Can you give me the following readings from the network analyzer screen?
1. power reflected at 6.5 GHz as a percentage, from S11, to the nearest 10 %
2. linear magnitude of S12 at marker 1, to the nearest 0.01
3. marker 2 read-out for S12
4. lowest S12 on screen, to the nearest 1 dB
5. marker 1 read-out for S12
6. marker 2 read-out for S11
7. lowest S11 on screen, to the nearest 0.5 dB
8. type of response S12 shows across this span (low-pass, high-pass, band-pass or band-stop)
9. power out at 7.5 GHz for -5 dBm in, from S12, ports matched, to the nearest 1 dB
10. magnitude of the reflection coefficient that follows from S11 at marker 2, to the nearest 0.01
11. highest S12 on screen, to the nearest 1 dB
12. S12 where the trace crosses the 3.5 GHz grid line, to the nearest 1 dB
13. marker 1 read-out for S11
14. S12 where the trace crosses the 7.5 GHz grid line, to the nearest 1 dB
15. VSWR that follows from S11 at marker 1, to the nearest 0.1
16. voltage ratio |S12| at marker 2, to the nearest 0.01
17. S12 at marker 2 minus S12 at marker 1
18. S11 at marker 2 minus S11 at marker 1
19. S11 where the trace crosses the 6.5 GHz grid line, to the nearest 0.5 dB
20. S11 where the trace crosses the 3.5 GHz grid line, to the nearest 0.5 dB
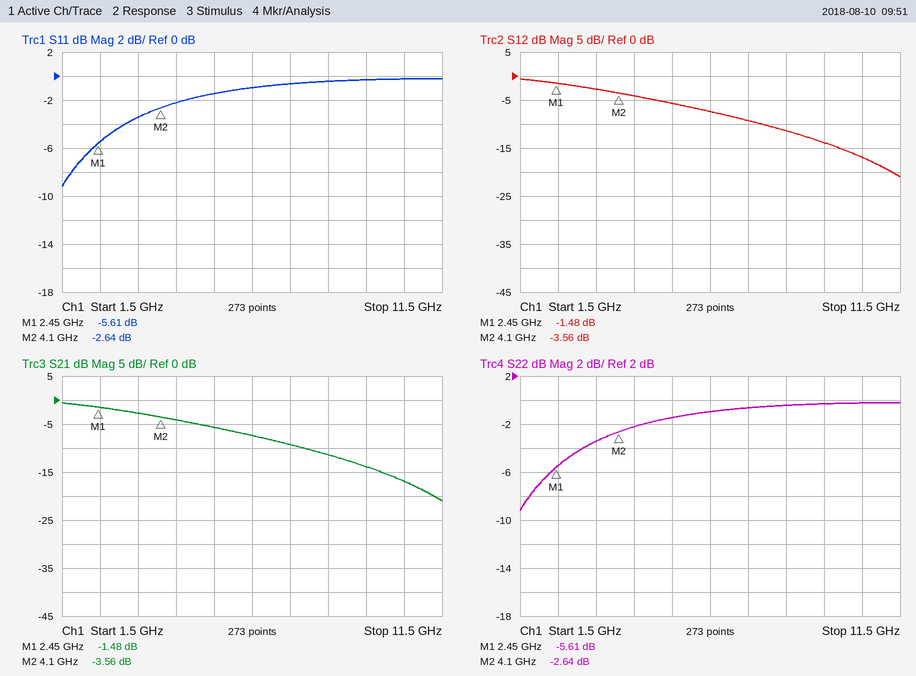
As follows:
80 %
0.84
-3.56 dB
-21 dB
-1.48 dB
-2.64 dB
-9.0 dB
low-pass
-14 dBm
0.74
-1 dB
-3 dB
-5.61 dB
-9 dB
3.2
0.66
-2.08 dB
2.97 dB
-1.0 dB
-3.5 dB
